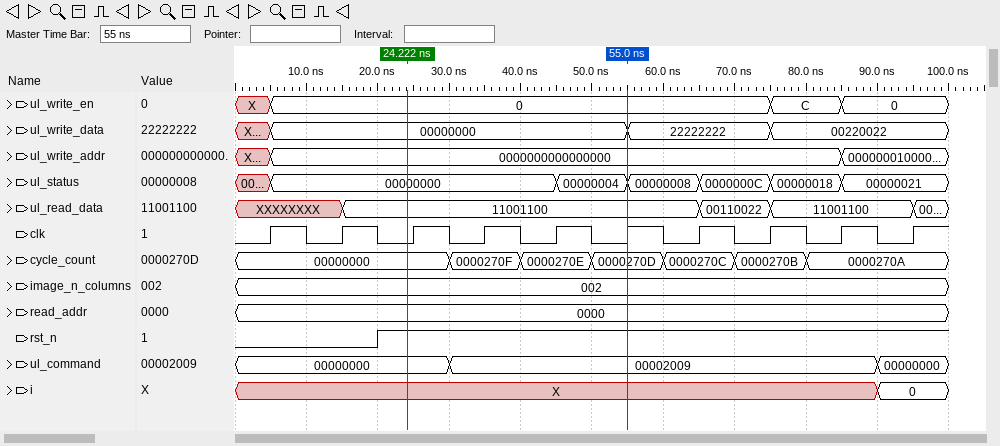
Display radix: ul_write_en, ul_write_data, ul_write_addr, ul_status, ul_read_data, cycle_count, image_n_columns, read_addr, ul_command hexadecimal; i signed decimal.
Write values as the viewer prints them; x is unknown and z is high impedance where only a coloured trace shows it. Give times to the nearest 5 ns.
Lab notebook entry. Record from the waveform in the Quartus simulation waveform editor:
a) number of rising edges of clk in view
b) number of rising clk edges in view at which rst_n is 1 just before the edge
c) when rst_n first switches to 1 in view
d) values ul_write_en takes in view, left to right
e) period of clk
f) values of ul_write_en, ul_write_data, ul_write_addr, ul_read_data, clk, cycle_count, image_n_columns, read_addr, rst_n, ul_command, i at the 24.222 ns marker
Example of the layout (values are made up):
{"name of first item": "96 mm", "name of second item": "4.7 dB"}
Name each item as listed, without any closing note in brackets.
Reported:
{"number of rising edges of clk in view": "10", "number of rising clk edges in view at which rst_n is 1 just before the edge": "8", "when rst_n first switches to 1 in view": "20 ns", "values ul_write_en takes in view, left to right": "X, 0, C, 0", "period of clk": "10 ns", "values of ul_write_en, ul_write_data, ul_write_addr, ul_read_data, clk, cycle_count, image_n_columns, read_addr, rst_n, ul_command, i at the 24.222 ns marker": "ul_write_en=0, ul_write_data=00000000, ul_write_addr=0000000000000000, ul_read_data=11001100, clk=0, cycle_count=00000000, image_n_columns=002, read_addr=0000, rst_n=1, ul_command=00000000, i=X"}
